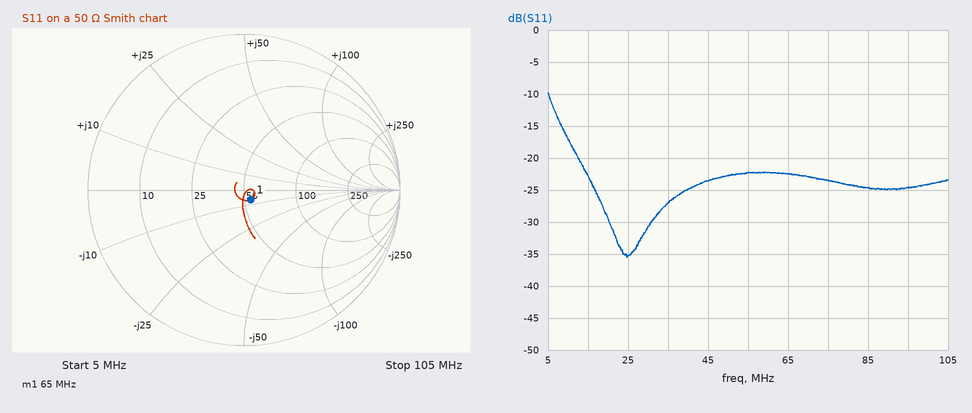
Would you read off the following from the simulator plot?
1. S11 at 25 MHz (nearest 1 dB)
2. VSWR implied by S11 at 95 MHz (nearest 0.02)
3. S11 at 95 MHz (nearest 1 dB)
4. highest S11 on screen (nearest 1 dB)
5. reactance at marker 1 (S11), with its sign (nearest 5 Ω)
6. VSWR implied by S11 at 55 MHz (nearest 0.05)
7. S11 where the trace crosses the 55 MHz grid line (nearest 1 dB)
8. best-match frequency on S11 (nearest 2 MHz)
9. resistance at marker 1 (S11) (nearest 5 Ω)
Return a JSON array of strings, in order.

["-35 dB", "1.12", "-25 dB", "-10 dB", "-5 Ω", "1.15", "-22 dB", "24 MHz", "55 Ω"]
